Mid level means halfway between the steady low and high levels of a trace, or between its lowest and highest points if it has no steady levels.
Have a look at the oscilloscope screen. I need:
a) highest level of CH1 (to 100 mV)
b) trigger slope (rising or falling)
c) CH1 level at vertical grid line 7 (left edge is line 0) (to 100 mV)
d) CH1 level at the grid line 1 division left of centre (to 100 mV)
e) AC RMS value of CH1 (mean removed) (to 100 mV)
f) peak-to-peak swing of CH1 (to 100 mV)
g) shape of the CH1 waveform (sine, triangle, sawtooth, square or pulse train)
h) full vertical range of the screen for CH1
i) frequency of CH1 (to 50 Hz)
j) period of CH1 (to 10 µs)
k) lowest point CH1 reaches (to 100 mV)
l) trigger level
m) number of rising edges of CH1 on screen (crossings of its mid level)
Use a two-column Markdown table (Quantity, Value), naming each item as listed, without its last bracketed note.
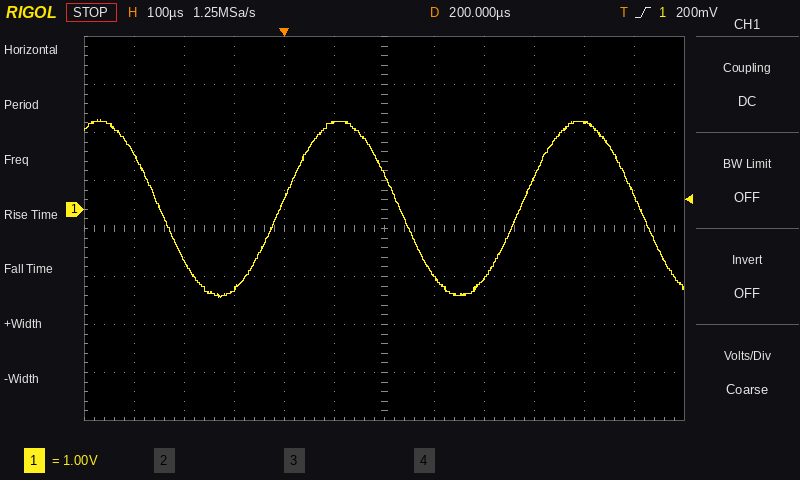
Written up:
| Quantity | Value |
|---|---|
| highest level of CH1 | 1.9 V |
| trigger slope | rising |
| CH1 level at vertical grid line 7 (left edge is line 0) | -1.4 V |
| CH1 level at the grid line 1 division left of centre | 1.8 V |
| AC RMS value of CH1 (mean removed) | 1.3 V |
| peak-to-peak swing of CH1 | 3.7 V |
| shape of the CH1 waveform | sine |
| full vertical range of the screen for CH1 | 8 V |
| frequency of CH1 | 2.10 kHz |
| period of CH1 | 480 µs |
| lowest point CH1 reaches | -1.8 V |
| trigger level | 200 mV |
| number of rising edges of CH1 on screen | 2 |
